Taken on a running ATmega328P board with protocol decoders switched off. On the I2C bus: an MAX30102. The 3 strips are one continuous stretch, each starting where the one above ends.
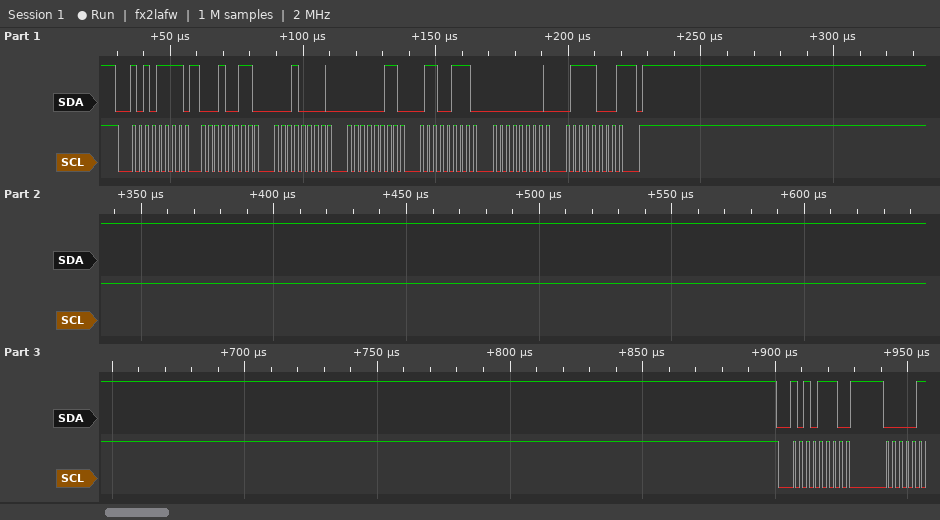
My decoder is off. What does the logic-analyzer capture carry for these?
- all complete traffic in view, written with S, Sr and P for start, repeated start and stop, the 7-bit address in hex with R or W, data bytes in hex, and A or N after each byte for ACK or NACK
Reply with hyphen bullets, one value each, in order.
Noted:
- S 57R A 13 A 10 A 03 A 67 A 00 A 78 N P S 57W A
